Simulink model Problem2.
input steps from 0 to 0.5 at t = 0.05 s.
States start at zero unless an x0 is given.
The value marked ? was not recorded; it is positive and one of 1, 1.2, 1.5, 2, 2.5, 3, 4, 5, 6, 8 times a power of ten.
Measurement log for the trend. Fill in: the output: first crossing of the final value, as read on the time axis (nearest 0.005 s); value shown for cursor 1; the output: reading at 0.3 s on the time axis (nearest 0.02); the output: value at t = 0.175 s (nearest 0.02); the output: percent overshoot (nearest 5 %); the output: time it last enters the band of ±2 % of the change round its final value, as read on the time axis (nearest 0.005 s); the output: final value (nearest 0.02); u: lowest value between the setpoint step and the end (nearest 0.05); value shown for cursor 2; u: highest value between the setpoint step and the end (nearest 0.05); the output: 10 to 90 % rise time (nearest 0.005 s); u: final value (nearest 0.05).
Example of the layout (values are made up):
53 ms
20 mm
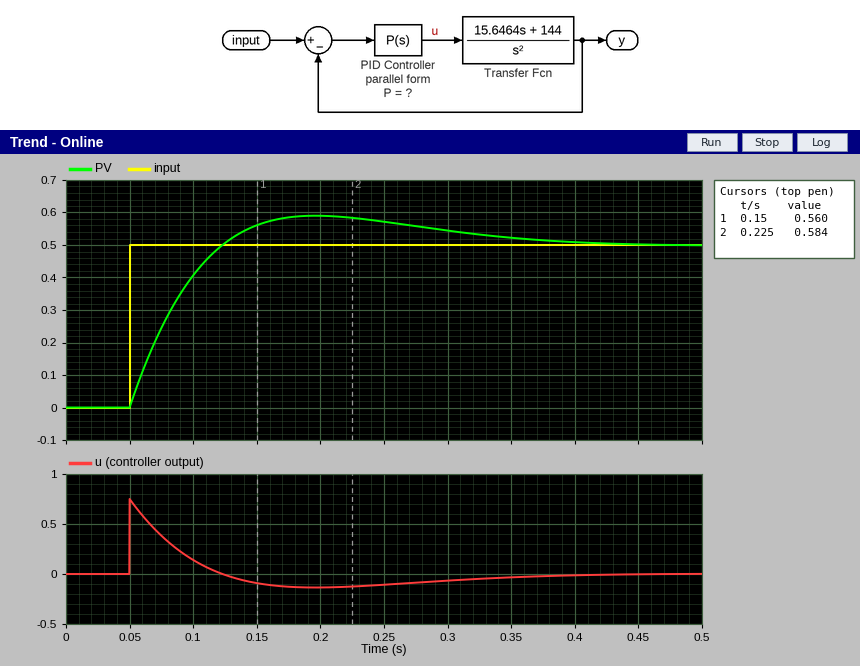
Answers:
0.125 s
0.560
0.54
0.58
20 %
0.395 s
0.50
-0.15
0.584
0.75
0.055 s
0.00
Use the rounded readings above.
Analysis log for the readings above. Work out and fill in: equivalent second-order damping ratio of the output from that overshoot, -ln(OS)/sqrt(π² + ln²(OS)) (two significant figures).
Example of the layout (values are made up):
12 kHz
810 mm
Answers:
0.46
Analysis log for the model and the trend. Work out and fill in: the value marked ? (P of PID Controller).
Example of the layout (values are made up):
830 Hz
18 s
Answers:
1.5
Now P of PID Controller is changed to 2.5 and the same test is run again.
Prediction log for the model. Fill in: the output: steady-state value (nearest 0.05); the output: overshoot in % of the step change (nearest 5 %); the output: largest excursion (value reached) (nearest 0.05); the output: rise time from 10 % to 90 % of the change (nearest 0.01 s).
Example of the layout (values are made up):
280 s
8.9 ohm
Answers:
0.50
15 %
0.55
0.04 s
